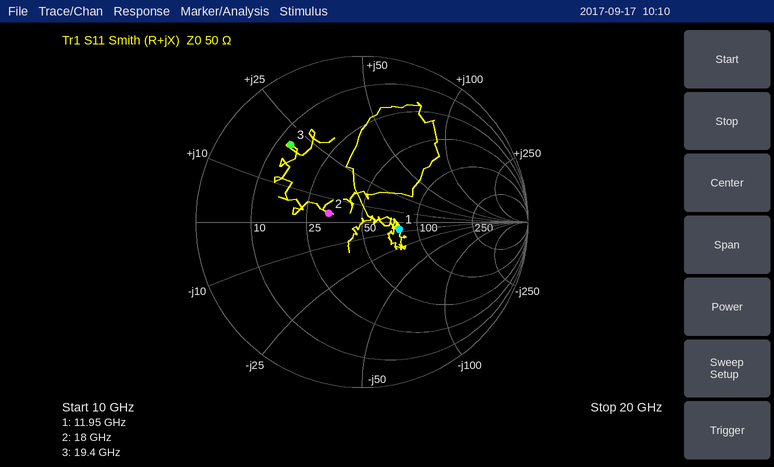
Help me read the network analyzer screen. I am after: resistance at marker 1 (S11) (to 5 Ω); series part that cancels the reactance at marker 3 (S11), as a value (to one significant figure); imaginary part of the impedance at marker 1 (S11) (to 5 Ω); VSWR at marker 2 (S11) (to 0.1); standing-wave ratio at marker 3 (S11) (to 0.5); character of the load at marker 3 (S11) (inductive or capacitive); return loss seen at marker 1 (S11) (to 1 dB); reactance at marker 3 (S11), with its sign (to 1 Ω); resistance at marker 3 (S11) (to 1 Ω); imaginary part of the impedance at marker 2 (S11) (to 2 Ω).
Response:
80 Ω
400 fF
-5 Ω
1.5
4.5
inductive
13 dB
+21 Ω
13 Ω
+4 Ω
